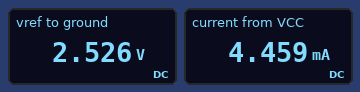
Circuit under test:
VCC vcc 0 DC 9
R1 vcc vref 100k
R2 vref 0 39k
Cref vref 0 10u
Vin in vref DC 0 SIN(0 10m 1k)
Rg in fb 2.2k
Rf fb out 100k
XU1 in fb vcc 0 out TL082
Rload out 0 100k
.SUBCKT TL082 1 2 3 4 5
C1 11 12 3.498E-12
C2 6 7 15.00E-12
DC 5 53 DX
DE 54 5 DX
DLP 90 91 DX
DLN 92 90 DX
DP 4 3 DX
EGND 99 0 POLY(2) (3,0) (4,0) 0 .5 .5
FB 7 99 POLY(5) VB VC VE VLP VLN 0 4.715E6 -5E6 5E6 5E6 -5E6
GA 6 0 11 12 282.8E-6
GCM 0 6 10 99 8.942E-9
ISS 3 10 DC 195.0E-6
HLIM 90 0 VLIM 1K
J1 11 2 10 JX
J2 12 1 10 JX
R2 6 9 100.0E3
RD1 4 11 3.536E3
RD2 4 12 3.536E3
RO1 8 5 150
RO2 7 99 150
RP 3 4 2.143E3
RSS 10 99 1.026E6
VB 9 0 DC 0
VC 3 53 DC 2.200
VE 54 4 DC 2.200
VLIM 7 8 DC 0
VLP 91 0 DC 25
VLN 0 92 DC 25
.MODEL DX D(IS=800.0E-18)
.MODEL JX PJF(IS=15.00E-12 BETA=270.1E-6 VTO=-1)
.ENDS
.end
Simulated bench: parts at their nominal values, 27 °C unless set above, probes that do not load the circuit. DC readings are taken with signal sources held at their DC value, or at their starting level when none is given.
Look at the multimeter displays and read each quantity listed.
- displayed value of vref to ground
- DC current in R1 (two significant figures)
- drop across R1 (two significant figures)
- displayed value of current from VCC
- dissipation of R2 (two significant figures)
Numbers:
2.526 V
65 µA
6.5 V
4.459 mA
160 µW
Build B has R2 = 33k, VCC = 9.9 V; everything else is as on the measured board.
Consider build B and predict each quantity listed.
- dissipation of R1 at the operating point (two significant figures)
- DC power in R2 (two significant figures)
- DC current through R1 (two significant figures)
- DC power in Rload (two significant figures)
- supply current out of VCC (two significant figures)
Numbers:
550 µW
180 µW
74 µA
61 µW
4.9 mA
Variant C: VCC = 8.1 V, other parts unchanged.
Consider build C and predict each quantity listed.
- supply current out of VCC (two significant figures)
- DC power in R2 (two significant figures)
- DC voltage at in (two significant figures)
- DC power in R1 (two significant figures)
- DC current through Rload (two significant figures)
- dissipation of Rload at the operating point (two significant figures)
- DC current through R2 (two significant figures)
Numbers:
4.0 mA
130 µW
2.3 V
340 µW
23 µA
52 µW
58 µA
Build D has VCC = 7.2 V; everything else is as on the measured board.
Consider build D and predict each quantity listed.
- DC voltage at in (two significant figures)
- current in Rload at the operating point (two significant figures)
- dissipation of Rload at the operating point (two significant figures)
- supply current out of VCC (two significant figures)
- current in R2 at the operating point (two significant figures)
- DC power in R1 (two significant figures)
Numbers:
2.0 V
20 µA
41 µW
3.6 mA
52 µA
270 µW
